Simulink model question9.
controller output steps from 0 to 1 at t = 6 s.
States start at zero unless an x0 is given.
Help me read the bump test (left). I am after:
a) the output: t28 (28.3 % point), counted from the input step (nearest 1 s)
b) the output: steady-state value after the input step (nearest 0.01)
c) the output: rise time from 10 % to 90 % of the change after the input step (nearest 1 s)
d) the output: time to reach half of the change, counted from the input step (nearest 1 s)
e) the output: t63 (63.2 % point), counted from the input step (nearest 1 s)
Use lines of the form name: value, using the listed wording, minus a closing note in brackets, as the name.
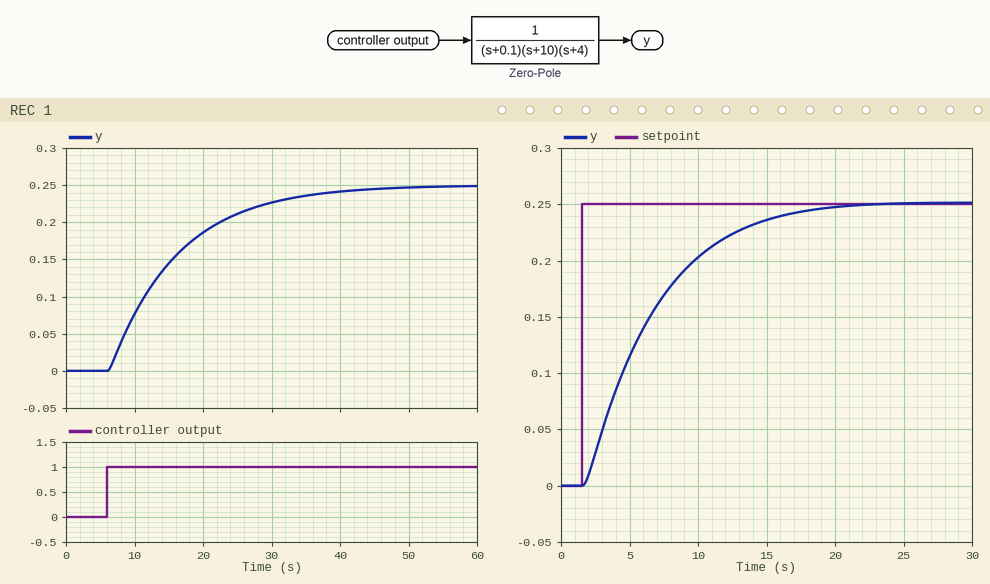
the output: t28 (28.3 % point), counted from the input step: 4 s
the output: steady-state value after the input step: 0.25
the output: rise time from 10 % to 90 % of the change after the input step: 22 s
the output: time to reach half of the change, counted from the input step: 7 s
the output: t63 (63.2 % point), counted from the input step: 10 s
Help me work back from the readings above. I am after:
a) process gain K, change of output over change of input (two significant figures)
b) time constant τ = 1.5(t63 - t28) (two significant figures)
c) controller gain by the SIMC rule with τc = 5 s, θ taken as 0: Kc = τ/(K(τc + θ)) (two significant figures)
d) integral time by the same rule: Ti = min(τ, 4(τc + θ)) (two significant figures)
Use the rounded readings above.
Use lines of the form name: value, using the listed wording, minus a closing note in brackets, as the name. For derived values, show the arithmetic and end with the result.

process gain K, change of output over change of input: (0.25 - 0) / 1 = 0.25
time constant τ = 1.5(t63 - t28): 1.5 × (10 - 4) = 9.0 s
controller gain by the SIMC rule with τc = 5 s, θ taken as 0: Kc = τ/(K(τc + θ)): 9 / (0.25 × (5 + 0)) = 7.2
integral time by the same rule: Ti = min(τ, 4(τc + θ)): min(9, 4 × (5 + 0)) = 9.0 s
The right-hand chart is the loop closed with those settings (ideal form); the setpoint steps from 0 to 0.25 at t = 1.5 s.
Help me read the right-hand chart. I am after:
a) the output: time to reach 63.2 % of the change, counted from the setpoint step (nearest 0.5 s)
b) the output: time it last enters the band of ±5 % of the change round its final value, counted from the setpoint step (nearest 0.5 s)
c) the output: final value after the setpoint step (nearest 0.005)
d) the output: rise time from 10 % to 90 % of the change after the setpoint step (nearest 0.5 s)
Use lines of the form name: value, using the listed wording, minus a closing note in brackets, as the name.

the output: time to reach 63.2 % of the change, counted from the setpoint step: 5.5 s
the output: time it last enters the band of ±5 % of the change round its final value, counted from the setpoint step: 14.0 s
the output: final value after the setpoint step: 0.250
the output: rise time from 10 % to 90 % of the change after the setpoint step: 10.5 s
